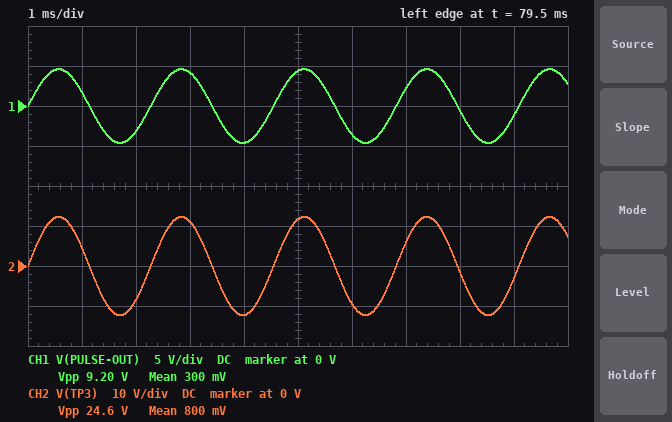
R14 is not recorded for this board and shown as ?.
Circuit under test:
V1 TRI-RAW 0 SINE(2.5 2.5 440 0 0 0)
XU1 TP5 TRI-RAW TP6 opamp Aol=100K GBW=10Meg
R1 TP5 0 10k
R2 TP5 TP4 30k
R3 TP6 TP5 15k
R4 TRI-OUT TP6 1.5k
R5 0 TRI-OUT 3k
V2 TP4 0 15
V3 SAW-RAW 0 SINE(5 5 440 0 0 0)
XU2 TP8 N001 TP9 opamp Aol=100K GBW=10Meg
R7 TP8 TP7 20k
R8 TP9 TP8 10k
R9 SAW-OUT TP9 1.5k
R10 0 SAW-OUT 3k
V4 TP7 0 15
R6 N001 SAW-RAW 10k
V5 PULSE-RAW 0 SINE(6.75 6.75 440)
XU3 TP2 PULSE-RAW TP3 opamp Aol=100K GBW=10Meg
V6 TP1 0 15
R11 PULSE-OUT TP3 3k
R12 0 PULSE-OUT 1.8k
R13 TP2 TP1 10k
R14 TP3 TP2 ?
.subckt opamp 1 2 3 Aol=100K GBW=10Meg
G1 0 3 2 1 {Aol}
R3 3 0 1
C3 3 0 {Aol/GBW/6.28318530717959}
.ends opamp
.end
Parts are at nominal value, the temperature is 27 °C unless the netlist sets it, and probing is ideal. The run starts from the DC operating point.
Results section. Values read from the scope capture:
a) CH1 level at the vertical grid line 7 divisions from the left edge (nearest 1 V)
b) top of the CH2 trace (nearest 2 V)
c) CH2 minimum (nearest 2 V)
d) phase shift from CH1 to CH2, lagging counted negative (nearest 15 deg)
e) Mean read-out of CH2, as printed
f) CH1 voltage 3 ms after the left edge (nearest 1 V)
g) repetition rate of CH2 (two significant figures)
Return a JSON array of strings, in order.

["2 V", "12 V", "-12 V", "0 deg", "800 mV", "4 V", "440 Hz"]
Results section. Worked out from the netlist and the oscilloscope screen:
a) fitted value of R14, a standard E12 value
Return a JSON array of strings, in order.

["8.2 kΩ"]
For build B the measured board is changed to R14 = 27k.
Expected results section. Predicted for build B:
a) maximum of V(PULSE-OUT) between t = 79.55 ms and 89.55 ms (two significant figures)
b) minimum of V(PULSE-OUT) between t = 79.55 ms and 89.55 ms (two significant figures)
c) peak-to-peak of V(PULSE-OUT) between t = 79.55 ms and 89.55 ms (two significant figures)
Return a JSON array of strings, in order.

["3.5 V", "-15 V", "19 V"]
